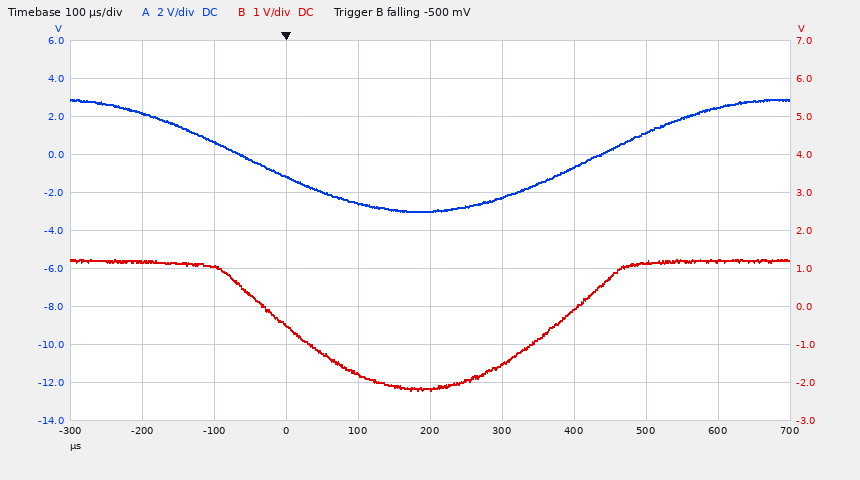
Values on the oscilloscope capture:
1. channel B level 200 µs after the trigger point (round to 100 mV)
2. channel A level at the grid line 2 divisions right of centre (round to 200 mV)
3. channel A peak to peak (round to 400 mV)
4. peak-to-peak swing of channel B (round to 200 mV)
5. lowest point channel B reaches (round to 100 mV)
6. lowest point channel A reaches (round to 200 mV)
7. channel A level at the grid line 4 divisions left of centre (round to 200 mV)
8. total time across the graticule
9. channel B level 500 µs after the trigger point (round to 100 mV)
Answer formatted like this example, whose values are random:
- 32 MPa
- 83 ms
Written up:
- -2.2 V
- -600 mV
- 6.0 V
- 3.4 V
- -2.2 V
- -3.0 V
- 2.2 V
- 1 ms
- 1.2 V
